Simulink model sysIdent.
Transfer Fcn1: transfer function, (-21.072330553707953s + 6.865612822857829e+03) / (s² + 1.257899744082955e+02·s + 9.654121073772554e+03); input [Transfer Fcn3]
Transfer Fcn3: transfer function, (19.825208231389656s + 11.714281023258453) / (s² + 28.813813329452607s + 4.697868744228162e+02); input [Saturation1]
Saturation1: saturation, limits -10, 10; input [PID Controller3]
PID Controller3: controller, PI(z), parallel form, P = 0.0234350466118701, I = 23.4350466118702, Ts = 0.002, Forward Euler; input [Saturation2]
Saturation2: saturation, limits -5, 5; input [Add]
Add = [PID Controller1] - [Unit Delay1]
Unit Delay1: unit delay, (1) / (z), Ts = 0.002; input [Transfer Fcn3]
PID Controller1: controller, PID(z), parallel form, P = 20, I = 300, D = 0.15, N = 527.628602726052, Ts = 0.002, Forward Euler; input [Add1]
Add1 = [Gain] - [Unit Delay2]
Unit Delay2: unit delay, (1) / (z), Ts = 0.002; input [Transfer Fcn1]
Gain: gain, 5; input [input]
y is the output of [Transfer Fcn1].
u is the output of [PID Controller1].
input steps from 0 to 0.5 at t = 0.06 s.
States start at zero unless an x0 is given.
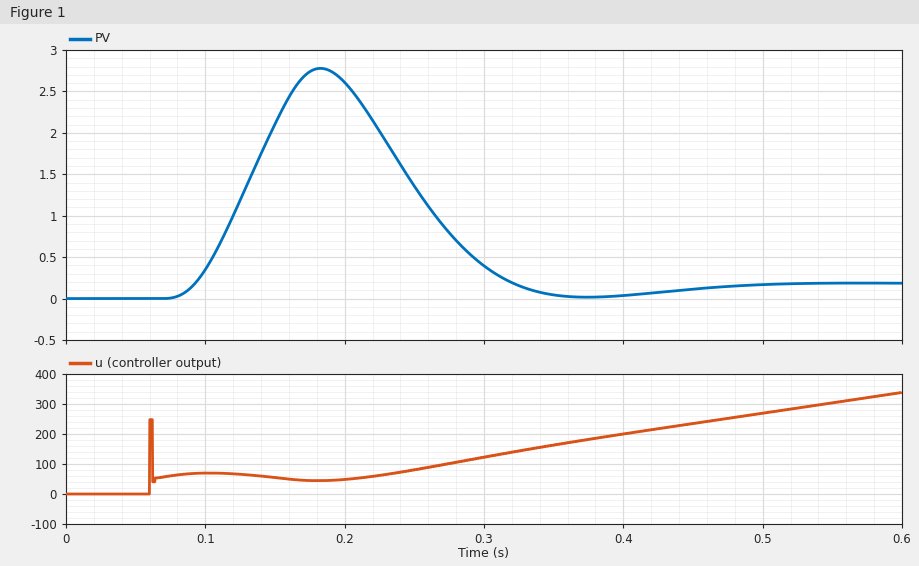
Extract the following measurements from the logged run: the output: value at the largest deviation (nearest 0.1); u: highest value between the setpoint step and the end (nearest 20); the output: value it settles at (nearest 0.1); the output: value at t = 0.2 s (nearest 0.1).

2.8
340
0.2
2.6
